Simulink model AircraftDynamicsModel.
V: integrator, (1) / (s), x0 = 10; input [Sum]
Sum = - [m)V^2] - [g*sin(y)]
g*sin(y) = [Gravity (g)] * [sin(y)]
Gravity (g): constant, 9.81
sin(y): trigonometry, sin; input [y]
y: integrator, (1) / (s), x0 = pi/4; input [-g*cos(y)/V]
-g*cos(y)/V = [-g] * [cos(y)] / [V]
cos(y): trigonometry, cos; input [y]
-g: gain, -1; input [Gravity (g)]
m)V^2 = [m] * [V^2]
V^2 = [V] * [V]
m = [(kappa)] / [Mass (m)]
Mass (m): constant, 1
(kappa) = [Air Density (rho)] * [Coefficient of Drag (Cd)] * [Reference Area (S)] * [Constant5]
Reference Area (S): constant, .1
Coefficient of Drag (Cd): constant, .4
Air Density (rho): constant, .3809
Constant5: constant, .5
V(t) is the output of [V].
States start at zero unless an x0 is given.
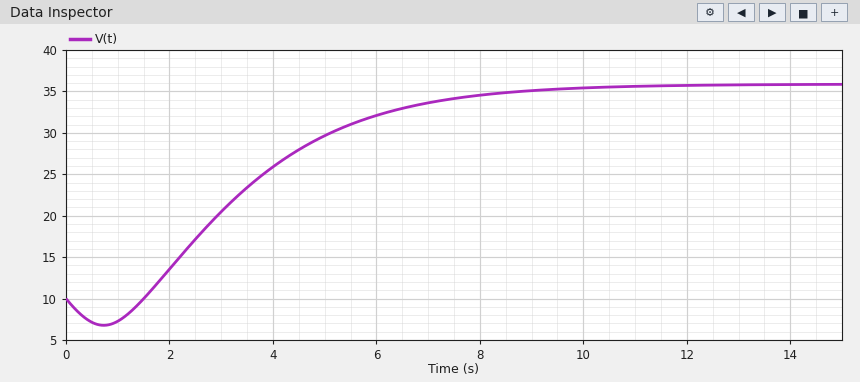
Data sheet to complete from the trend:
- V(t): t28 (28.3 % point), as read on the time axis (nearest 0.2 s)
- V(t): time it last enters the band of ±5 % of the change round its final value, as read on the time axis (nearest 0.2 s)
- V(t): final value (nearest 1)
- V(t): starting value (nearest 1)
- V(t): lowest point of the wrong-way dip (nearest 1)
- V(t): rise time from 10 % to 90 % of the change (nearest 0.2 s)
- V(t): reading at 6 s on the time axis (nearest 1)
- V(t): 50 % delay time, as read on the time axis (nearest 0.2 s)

2.6 s
8.0 s
36
10
7
4.8 s
32
3.4 s
